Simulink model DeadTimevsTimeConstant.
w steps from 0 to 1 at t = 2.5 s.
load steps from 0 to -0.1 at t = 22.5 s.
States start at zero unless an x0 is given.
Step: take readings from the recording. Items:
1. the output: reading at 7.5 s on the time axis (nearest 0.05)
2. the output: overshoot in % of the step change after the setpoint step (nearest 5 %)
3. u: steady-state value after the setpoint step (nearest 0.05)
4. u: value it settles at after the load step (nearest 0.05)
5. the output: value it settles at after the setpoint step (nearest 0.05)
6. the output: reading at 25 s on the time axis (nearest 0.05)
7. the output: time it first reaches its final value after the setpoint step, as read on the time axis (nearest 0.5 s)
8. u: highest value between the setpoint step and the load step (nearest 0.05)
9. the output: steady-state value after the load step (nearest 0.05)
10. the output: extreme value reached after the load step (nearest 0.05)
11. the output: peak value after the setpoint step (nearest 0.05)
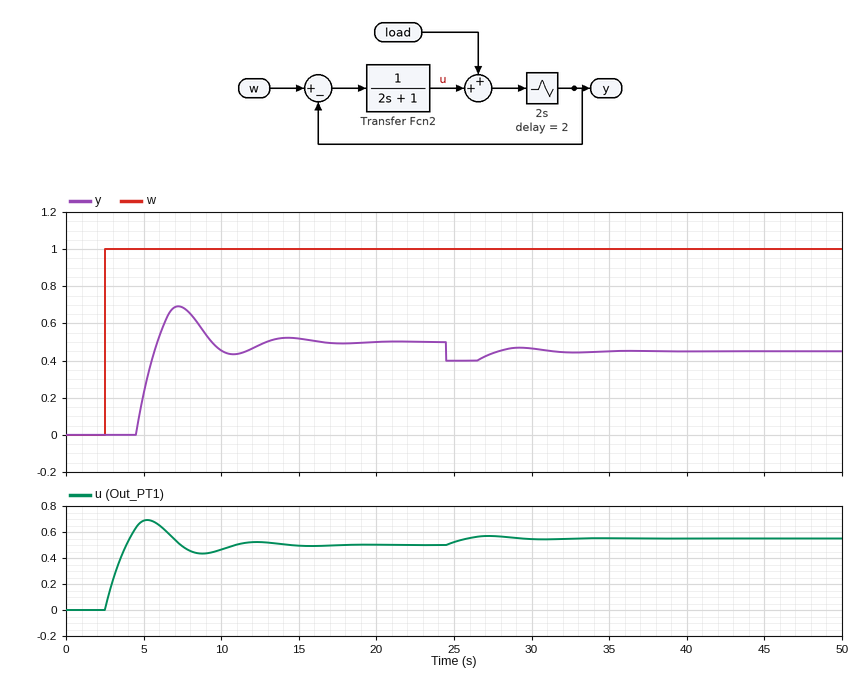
0.70
40 %
0.50
0.55
0.50
0.40
6.0 s
0.70
0.45
0.40
0.70
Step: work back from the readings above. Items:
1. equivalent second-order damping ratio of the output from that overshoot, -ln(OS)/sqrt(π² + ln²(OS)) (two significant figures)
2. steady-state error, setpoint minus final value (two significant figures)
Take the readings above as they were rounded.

0.28
0.50
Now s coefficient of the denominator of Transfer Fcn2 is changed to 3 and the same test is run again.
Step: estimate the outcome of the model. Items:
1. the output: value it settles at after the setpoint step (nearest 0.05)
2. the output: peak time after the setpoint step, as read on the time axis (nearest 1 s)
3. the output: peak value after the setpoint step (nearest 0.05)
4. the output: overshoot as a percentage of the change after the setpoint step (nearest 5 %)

0.50
8 s
0.60
20 %
